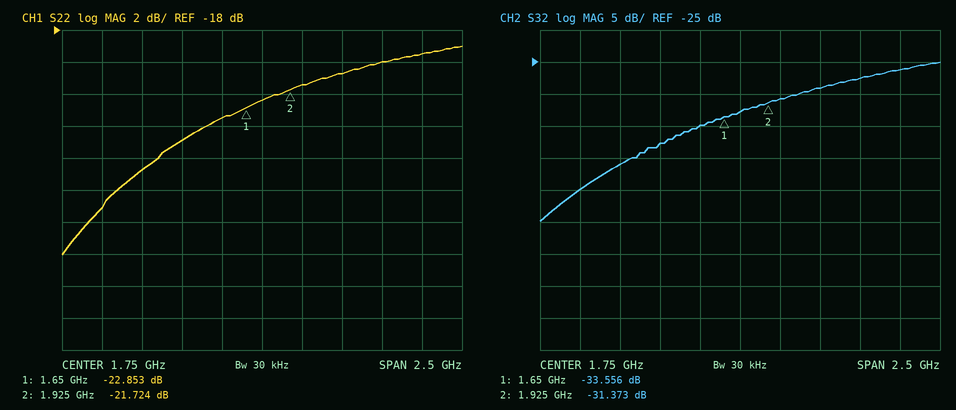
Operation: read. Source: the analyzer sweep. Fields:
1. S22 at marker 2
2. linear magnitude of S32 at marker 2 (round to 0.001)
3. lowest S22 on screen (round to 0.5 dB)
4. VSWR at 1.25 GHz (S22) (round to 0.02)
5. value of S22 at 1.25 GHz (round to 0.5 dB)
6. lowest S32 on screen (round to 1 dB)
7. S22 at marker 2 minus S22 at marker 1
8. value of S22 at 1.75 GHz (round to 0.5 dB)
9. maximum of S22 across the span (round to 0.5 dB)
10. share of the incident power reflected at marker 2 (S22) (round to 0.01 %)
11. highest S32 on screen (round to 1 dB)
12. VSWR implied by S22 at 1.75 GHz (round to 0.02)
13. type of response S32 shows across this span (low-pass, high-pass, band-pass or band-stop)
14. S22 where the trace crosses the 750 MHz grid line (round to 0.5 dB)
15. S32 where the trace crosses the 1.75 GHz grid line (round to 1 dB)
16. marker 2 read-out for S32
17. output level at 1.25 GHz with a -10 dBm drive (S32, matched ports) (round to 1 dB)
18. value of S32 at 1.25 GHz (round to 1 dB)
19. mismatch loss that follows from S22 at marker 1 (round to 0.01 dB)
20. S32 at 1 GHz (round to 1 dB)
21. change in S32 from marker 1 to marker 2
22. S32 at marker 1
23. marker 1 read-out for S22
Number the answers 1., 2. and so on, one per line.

1. -21.724 dB
2. 0.027
3. -32.0 dB
4. 1.12
5. -25.0 dB
6. -50 dB
7. 1.129 dB
8. -22.5 dB
9. -19.0 dB
10. 0.67 %
11. -25 dB
12. 1.16
13. high-pass
14. -29.0 dB
15. -33 dB
16. -31.373 dB
17. -48 dBm
18. -38 dB
19. 0.02 dB
20. -41 dB
21. 2.183 dB
22. -33.556 dB
23. -22.853 dB
